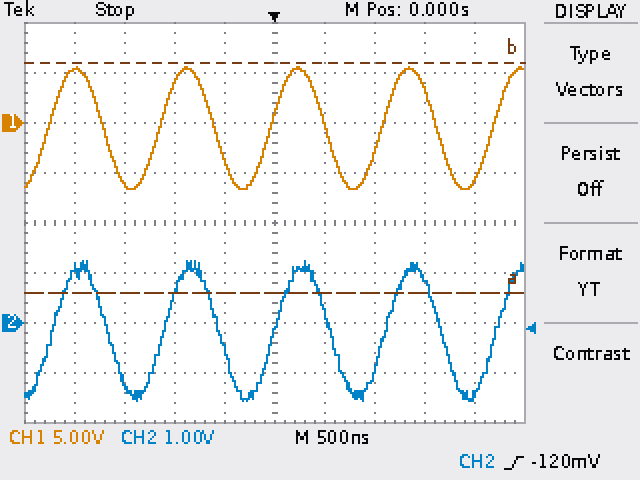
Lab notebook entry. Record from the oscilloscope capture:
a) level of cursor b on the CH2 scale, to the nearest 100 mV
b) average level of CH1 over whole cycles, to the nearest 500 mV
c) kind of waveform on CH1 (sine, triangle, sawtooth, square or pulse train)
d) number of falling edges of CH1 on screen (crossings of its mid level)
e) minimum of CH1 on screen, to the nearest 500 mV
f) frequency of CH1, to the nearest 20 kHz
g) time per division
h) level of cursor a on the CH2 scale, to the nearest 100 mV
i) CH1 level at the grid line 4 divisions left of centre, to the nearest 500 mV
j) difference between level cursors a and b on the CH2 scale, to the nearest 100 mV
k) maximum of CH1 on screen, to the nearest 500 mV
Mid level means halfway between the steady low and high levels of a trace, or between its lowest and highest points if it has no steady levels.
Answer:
5.2 V
-500 mV
sine
4
-6.5 V
900 kHz
500 ns
600 mV
5.5 V
4.6 V
5.5 V
